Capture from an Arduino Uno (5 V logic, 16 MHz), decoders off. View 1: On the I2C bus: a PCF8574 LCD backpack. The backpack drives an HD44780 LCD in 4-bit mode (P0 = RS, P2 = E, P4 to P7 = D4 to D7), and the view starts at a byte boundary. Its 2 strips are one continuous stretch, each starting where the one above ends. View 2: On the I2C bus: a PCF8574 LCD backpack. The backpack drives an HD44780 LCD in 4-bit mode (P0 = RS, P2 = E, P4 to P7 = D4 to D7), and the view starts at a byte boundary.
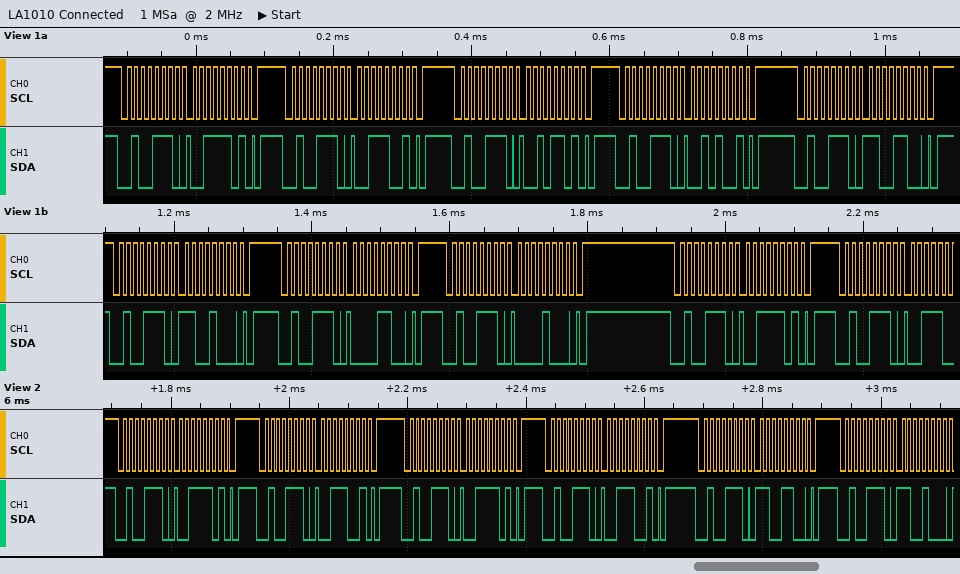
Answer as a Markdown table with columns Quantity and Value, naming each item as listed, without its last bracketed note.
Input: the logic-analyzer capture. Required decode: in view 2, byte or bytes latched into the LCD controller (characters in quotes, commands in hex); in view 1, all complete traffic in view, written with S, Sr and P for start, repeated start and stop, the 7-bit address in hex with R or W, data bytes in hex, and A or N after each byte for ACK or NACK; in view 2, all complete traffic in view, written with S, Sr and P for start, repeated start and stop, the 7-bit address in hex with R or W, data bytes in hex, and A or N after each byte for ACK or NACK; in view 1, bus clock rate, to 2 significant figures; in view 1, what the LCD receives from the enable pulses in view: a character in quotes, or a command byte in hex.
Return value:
| Quantity | Value |
|---|---|
| in view 2, byte or bytes latched into the LCD controller | '3' |
| in view 1, all complete traffic in view, written with S, Sr and P for start, repeated start and stop, the 7-bit address in hex with R or W, data bytes in hex, and A or N after each byte for ACK or NACK | S 27W A 3D A P S 27W A 39 A P S 27W A 2D A P S 27W A 29 A P S 27W A CC A P S 27W A C8 A P S 27W A 0C A P S 27W A 08 A P S 27W A 3D A P S 27W A |
| in view 2, all complete traffic in view, written with S, Sr and P for start, repeated start and stop, the 7-bit address in hex with R or W, data bytes in hex, and A or N after each byte for ACK or NACK | S 27W A 3D A P S 27W A 39 A P S 27W A 3D A P S 27W A 39 A P S 27W A CC A P S 27W A C8 A |
| in view 1, bus clock rate, to 2 significant figures | 100 kHz |
| in view 1, what the LCD receives from the enable pulses in view: a character in quotes, or a command byte in hex | '2' 0xC0 |
